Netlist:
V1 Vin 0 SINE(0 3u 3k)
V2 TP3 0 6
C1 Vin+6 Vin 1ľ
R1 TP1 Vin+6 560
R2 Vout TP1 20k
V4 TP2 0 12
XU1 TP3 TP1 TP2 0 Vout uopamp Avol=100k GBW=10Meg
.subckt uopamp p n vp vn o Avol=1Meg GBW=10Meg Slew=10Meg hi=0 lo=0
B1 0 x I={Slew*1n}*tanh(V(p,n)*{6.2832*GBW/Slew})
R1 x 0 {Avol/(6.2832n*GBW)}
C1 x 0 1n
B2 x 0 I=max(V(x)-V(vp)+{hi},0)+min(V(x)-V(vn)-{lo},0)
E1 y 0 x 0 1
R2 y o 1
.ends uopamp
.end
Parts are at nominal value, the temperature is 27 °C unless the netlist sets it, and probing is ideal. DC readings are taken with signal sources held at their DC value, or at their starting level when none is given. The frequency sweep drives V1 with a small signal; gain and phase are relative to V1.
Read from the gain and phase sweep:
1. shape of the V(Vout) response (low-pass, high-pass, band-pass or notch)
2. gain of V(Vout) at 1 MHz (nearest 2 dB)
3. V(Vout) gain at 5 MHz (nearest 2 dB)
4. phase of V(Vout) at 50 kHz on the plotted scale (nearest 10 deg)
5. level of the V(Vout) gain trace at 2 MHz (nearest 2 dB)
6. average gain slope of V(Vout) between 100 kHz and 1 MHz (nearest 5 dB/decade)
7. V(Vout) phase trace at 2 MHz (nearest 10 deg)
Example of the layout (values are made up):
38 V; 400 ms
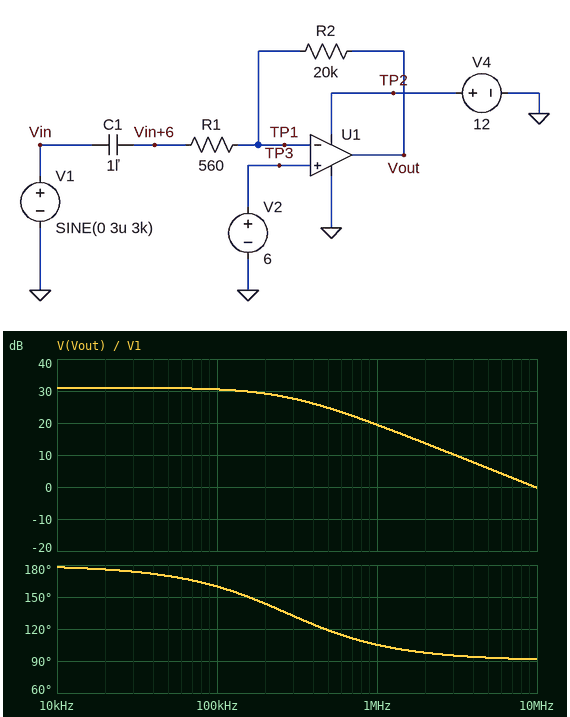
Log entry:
low-pass; 20 dB; 6 dB; 170 deg; 14 dB; -10 dB/decade; 100 deg
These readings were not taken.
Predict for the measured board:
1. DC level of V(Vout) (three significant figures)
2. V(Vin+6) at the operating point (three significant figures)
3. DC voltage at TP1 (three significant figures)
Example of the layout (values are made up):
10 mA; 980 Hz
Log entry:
6.00 V; 6.00 V; 6.00 V
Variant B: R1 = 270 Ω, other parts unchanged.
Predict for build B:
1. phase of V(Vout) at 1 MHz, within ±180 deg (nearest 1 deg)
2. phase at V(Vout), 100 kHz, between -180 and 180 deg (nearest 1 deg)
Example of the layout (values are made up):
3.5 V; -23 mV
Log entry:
98 deg; 143 deg
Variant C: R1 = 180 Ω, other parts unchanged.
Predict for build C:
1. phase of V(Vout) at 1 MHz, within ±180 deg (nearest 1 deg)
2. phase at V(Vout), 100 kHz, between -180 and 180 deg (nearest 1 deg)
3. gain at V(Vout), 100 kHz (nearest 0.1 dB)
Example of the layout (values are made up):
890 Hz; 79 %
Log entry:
95 deg; 132 deg; 37.4 dB
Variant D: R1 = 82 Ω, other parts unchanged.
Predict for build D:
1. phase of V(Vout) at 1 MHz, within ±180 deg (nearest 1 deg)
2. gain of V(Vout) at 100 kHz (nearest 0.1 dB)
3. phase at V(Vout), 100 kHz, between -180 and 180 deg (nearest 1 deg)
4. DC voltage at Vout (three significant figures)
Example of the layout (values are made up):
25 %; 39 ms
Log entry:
92 deg; 39.3 dB; 112 deg; 6.00 V
